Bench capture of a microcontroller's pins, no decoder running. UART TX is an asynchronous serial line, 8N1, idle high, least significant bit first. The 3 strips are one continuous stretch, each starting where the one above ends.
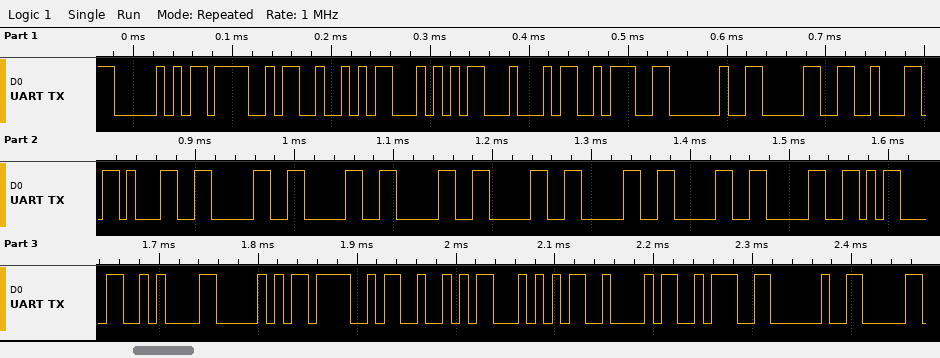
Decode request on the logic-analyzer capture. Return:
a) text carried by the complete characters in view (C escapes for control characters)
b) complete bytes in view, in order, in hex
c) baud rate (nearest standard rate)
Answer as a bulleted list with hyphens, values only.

- "PORTD: 0b10000000\r\nPORTB: "
- 50 4F 52 54 44 3A 20 30 62 31 30 30 30 30 30 30 30 0D 0A 50 4F 52 54 42 3A 20
- 115200 baud
